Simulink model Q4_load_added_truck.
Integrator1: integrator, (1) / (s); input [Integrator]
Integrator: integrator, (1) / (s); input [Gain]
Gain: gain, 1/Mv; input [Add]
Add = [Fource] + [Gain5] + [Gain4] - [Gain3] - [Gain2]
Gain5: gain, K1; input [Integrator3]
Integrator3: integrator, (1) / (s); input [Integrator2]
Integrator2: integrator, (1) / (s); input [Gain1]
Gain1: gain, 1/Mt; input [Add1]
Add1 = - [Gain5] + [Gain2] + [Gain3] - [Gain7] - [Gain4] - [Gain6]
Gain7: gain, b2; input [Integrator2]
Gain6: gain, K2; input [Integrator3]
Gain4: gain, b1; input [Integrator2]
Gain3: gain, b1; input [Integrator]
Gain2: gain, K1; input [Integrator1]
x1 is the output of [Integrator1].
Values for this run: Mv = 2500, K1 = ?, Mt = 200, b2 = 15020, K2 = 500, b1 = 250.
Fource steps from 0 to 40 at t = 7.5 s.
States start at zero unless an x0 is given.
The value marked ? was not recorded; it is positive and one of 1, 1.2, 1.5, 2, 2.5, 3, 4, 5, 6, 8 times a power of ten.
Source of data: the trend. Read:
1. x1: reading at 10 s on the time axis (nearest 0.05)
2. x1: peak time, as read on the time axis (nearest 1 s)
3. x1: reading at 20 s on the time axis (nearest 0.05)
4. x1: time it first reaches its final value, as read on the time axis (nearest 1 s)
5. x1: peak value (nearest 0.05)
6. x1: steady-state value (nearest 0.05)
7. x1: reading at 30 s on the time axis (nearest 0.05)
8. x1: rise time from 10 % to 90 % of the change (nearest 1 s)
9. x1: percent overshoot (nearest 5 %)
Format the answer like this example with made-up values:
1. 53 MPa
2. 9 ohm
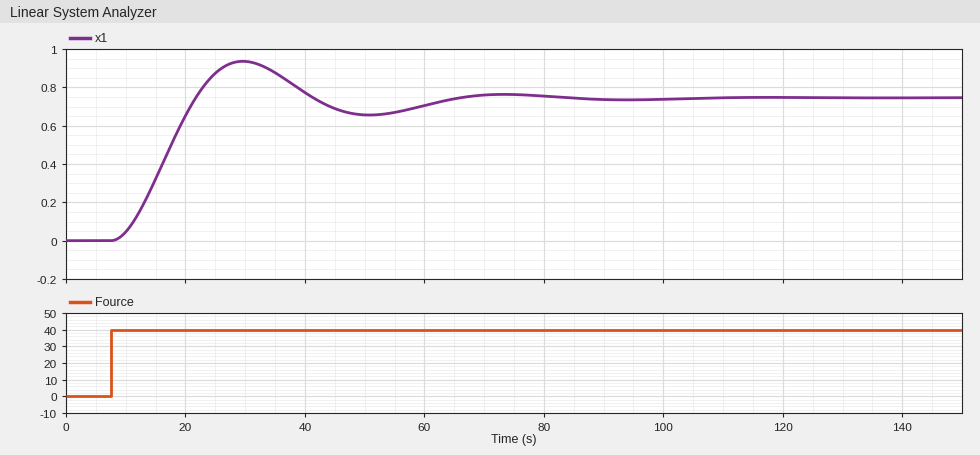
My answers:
1. 0.05
2. 30 s
3. 0.65
4. 22 s
5. 0.95
6. 0.75
7. 0.95
8. 10 s
9. 25 %
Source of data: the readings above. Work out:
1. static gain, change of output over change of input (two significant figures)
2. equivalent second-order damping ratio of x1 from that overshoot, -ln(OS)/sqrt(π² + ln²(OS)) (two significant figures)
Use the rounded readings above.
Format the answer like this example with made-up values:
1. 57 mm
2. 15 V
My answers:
1. 0.019
2. 0.40
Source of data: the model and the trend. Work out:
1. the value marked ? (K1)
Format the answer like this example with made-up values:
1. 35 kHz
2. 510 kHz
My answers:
1. 60
